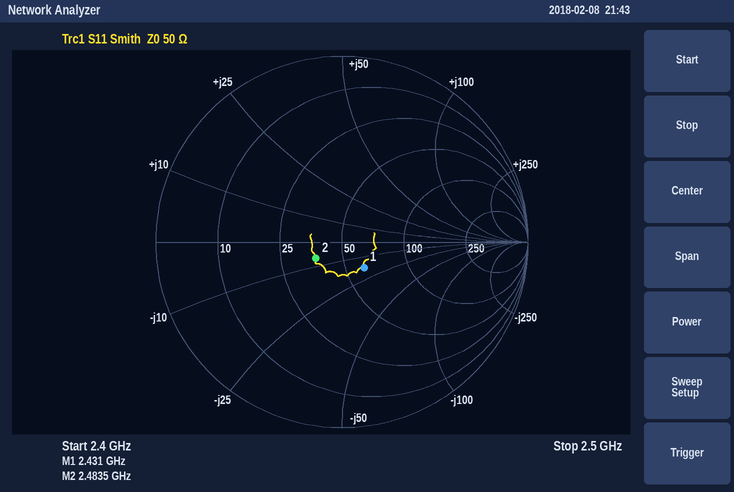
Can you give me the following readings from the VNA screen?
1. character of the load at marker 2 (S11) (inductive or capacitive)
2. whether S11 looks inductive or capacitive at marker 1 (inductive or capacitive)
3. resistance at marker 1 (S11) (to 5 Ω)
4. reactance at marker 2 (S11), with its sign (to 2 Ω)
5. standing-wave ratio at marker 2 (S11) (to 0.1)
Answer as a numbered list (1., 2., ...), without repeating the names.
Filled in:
1. capacitive
2. capacitive
3. 60 Ω
4. -6 Ω
5. 1.4
